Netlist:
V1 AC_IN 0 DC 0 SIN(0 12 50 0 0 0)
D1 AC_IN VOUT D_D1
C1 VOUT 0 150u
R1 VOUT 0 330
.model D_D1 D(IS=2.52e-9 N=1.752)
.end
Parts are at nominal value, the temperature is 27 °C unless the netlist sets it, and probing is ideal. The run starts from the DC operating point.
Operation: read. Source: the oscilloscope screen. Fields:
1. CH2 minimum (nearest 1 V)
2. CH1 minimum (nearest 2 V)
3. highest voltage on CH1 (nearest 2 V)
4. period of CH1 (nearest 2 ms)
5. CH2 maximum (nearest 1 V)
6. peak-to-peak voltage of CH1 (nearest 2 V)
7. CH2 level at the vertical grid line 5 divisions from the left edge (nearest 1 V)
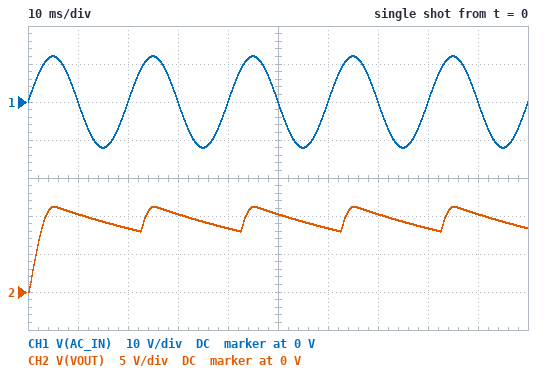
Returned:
0 V
-12 V
12 V
20 ms
11 V
24 V
10 V
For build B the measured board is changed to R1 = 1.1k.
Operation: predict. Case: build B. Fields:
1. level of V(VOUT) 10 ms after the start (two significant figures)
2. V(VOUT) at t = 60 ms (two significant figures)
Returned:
11 V
10 V
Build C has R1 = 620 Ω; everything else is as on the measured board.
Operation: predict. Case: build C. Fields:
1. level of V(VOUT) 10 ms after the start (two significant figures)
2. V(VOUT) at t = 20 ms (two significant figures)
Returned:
11 V
9.6 V
